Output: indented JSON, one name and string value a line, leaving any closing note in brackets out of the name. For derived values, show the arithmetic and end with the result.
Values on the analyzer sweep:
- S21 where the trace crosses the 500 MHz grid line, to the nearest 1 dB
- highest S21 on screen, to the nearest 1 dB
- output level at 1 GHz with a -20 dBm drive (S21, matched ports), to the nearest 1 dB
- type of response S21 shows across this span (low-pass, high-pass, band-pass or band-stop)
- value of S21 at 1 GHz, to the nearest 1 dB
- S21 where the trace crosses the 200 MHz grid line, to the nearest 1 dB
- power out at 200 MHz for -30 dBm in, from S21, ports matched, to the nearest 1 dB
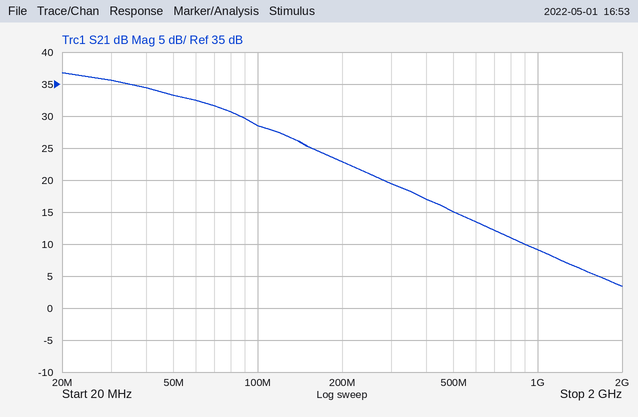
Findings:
{
  "S21 where the trace crosses the 500 MHz grid line, to the nearest 1 dB": "15 dB",
  "highest S21 on screen, to the nearest 1 dB": "37 dB",
  "output level at 1 GHz with a -20 dBm drive (S21, matched ports), to the nearest 1 dB": "-20 dBm + (9 dB) = -11 dBm",
  "type of response S21 shows across this span": "low-pass",
  "value of S21 at 1 GHz, to the nearest 1 dB": "9 dB",
  "S21 where the trace crosses the 200 MHz grid line, to the nearest 1 dB": "23 dB",
  "power out at 200 MHz for -30 dBm in, from S21, ports matched, to the nearest 1 dB": "-30 dBm + (23 dB) = -7 dBm"
}
